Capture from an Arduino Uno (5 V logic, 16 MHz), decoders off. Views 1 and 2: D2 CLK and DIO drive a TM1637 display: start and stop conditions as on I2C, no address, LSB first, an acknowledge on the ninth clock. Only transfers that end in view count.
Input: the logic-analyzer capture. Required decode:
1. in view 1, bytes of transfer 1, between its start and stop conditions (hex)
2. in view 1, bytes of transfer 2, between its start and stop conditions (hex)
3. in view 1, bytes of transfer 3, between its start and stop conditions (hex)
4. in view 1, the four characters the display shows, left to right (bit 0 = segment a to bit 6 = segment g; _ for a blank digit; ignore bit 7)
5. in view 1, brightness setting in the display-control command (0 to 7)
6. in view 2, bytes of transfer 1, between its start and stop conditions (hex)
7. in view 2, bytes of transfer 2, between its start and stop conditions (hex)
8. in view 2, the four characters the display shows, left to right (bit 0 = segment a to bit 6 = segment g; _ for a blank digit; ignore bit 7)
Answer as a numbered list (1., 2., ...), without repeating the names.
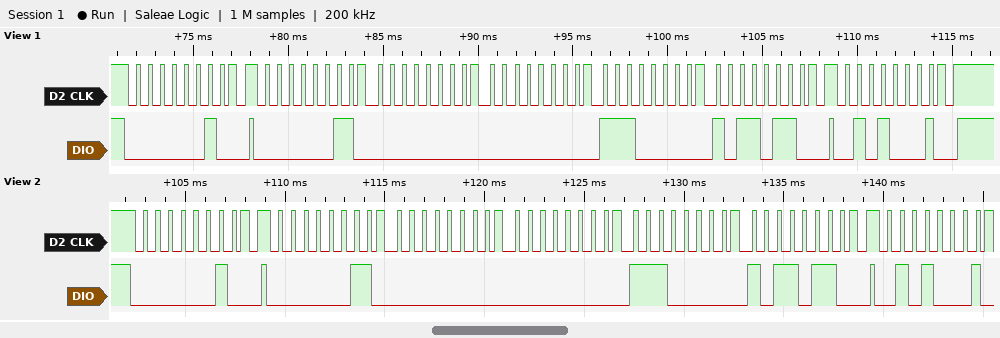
1. 40
2. C0 00 00 07 6D
3. 8A
4. __75
5. 2
6. 40
7. C0 00 00 07 6D
8. __75
